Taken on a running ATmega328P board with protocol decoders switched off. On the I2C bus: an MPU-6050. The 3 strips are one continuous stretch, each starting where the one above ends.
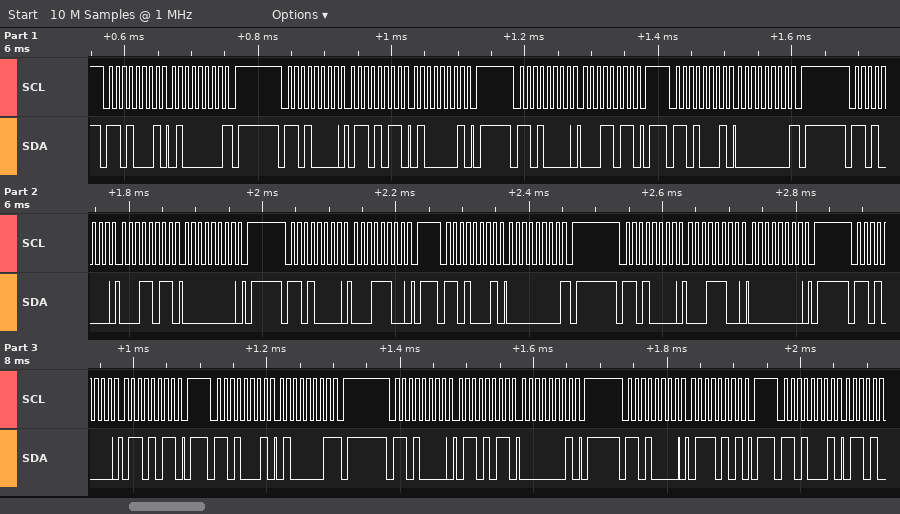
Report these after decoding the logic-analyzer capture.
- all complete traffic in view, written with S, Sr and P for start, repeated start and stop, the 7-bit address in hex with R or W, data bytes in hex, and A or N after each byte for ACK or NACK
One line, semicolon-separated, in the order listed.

S 68R A 40 N P S 68W A 6B A 41 A P S 68W A 1B A P S 68R A 00 N P S 68W A 1B A 00 A P S 68W A 1C A P S 68R A 00 N P S 68W A 1C A 00 A P S 68W A 6B A P S 68R A 41 N P S 68W A 6B A 01 A P S 68W A 75 A P S 68R A
